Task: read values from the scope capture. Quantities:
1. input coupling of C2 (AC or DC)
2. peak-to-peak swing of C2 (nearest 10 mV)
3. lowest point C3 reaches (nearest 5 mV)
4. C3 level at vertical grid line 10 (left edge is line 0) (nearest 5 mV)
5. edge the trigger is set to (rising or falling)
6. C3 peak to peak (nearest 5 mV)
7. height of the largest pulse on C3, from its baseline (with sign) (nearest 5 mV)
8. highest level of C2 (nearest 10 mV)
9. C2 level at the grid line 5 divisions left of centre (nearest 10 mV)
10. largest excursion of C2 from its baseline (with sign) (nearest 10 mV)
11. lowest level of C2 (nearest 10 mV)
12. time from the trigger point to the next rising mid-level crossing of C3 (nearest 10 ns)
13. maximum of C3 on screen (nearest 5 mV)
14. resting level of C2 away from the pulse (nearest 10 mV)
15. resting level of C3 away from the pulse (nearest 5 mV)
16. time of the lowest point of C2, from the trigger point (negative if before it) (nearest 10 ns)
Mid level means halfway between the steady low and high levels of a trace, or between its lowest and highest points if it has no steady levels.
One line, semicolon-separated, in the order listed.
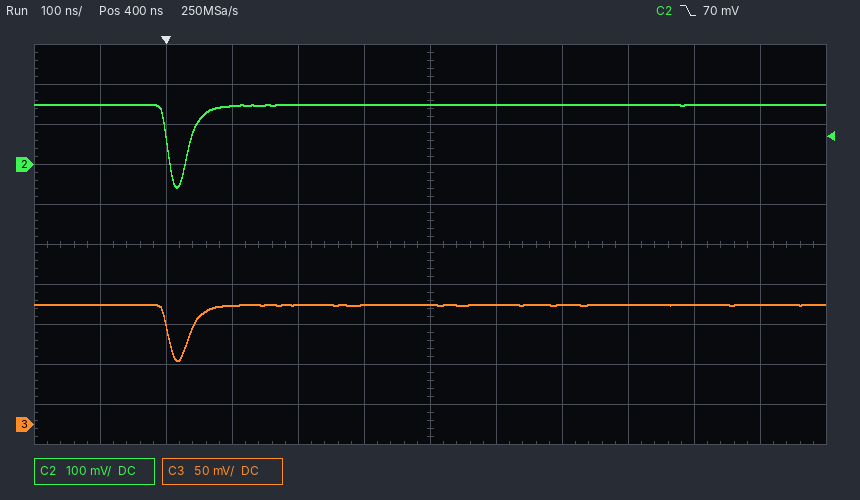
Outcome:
DC; 210 mV; 80 mV; 150 mV; falling; 70 mV; -70 mV; 150 mV; 150 mV; -210 mV; -60 mV; 40 ns; 150 mV; 150 mV; 150 mV; +20 ns
